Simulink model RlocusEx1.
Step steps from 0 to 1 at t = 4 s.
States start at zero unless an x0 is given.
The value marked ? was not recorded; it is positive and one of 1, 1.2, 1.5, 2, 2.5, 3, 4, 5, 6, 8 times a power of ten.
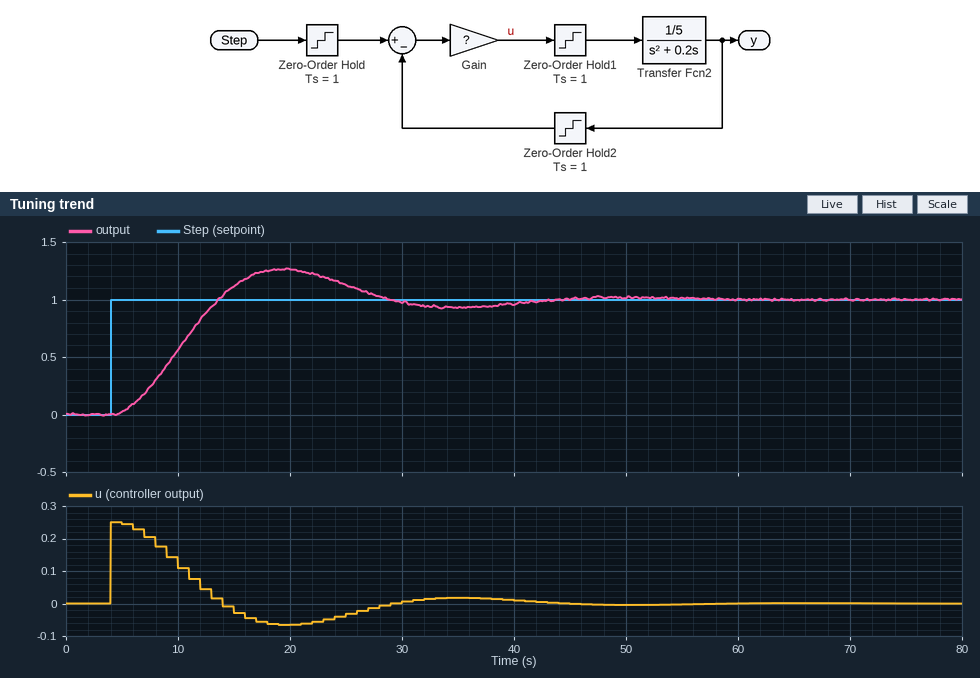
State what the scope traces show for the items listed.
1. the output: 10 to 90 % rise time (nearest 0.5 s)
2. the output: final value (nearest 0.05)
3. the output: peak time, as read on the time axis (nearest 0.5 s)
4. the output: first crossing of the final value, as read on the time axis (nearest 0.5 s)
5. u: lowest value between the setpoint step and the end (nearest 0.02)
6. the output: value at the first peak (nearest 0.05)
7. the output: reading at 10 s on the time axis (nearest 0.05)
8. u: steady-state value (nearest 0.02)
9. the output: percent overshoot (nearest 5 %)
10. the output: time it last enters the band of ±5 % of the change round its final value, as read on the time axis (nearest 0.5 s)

6.5 s
1.00
19.5 s
13.5 s
-0.06
1.25
0.55
0.00
25 %
38.5 s
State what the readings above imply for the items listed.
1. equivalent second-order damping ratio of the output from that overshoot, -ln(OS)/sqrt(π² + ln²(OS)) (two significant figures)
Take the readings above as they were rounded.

0.40
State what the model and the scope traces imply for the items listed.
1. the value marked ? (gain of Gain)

0.25
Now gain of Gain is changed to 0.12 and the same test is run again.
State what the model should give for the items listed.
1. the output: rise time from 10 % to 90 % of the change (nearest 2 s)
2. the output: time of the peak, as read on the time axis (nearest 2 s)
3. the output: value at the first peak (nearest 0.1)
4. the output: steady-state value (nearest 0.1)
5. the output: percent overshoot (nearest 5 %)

12 s
30 s
1.1
1.0
10 %
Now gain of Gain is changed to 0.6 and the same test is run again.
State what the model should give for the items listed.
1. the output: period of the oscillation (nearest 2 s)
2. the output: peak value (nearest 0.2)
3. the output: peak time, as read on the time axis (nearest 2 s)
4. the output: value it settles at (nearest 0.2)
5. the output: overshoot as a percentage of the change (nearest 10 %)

18 s
1.6
14 s
1.0
50 %
